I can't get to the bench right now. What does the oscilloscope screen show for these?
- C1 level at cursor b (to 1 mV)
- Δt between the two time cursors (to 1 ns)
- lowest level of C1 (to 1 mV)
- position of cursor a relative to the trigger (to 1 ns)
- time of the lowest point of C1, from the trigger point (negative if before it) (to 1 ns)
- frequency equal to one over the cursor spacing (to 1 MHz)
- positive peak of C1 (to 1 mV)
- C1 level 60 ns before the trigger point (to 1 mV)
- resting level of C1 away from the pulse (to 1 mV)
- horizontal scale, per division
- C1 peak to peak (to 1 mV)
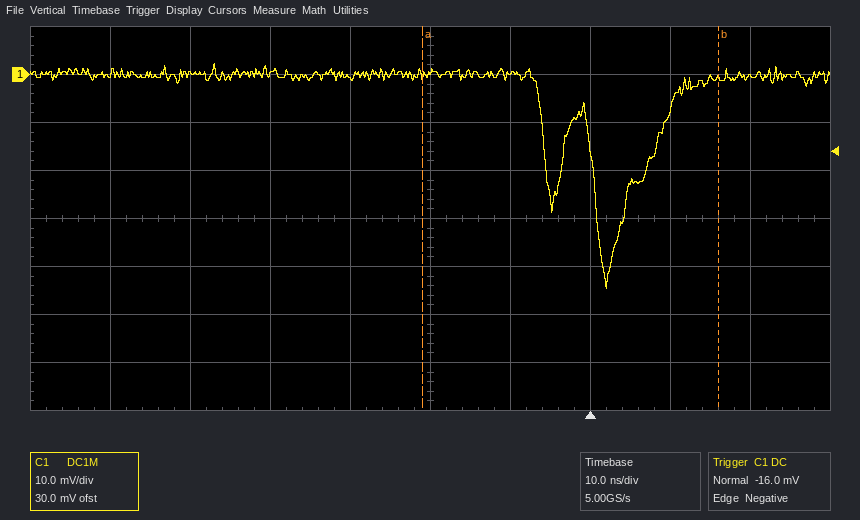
-1 mV
37 ns
-45 mV
-21 ns
+2 ns
27 MHz
2 mV
0 mV
0 mV
10 ns
47 mV
